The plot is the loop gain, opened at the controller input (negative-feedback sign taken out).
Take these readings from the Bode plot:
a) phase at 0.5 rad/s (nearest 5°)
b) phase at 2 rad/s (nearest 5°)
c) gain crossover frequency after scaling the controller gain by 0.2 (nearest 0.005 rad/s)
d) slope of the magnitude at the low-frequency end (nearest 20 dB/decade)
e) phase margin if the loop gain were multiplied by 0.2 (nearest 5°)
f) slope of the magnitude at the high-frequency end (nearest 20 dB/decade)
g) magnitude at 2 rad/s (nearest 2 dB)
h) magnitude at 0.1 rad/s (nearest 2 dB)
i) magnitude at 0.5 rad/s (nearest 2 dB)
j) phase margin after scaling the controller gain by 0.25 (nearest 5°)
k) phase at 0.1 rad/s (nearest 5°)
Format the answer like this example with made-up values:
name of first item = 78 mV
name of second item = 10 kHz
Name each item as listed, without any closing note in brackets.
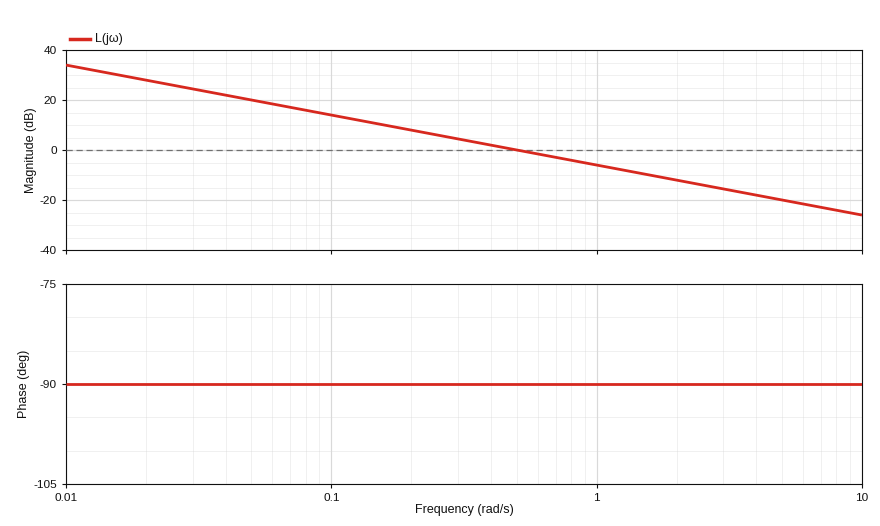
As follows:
phase at 0.5 rad/s = -90°
phase at 2 rad/s = -90°
gain crossover frequency after scaling the controller gain by 0.2 = 0.100 rad/s
slope of the magnitude at the low-frequency end = -20 dB/decade
phase margin if the loop gain were multiplied by 0.2 = 90°
slope of the magnitude at the high-frequency end = -20 dB/decade
magnitude at 2 rad/s = -12 dB
magnitude at 0.1 rad/s = 14 dB
magnitude at 0.5 rad/s = 0 dB
phase margin after scaling the controller gain by 0.25 = 90°
phase at 0.1 rad/s = -90°
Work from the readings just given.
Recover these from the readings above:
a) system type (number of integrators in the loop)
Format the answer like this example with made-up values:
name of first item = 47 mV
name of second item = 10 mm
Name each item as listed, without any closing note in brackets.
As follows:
system type = 1
